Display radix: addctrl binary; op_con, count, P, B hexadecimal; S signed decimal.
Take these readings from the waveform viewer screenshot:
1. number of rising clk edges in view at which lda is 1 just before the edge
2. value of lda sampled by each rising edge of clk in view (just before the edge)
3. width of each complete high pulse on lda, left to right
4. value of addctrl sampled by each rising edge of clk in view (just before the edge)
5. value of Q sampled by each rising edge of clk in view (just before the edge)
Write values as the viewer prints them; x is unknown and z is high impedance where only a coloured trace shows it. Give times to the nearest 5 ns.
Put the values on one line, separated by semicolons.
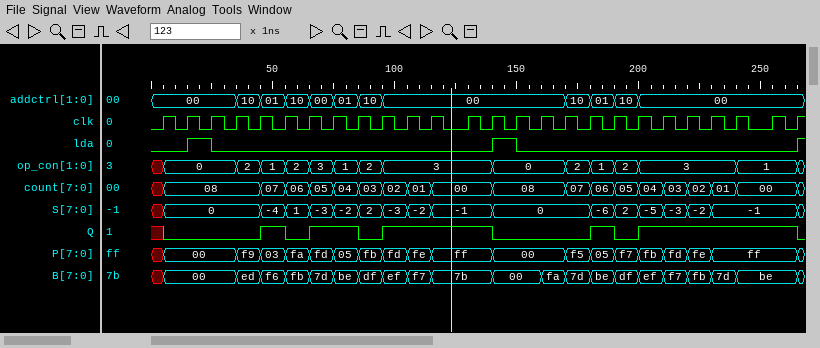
2; 0 0 1 0 0 0 0 0 0 0 0 0 0 0 1 0 0 0 0 0 0 0 0 0 0 0; 10 ns, 10 ns; 00, 00, 00, 00, 10, 01, 10, 00, 01, 10, 00, 00, 00, 00, 00, 00, 00, 10, 01, 10, 00, 00, 00, 00, 00, 00; x 0 0 0 0 1 0 1 1 0 1 1 1 1 0 0 0 0 1 0 1 1 1 1 1 1
